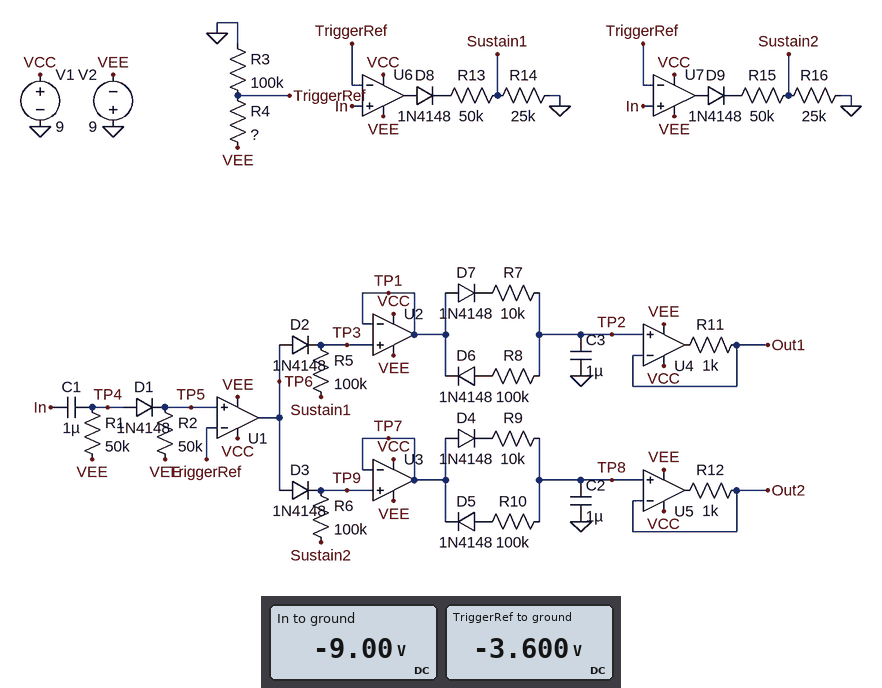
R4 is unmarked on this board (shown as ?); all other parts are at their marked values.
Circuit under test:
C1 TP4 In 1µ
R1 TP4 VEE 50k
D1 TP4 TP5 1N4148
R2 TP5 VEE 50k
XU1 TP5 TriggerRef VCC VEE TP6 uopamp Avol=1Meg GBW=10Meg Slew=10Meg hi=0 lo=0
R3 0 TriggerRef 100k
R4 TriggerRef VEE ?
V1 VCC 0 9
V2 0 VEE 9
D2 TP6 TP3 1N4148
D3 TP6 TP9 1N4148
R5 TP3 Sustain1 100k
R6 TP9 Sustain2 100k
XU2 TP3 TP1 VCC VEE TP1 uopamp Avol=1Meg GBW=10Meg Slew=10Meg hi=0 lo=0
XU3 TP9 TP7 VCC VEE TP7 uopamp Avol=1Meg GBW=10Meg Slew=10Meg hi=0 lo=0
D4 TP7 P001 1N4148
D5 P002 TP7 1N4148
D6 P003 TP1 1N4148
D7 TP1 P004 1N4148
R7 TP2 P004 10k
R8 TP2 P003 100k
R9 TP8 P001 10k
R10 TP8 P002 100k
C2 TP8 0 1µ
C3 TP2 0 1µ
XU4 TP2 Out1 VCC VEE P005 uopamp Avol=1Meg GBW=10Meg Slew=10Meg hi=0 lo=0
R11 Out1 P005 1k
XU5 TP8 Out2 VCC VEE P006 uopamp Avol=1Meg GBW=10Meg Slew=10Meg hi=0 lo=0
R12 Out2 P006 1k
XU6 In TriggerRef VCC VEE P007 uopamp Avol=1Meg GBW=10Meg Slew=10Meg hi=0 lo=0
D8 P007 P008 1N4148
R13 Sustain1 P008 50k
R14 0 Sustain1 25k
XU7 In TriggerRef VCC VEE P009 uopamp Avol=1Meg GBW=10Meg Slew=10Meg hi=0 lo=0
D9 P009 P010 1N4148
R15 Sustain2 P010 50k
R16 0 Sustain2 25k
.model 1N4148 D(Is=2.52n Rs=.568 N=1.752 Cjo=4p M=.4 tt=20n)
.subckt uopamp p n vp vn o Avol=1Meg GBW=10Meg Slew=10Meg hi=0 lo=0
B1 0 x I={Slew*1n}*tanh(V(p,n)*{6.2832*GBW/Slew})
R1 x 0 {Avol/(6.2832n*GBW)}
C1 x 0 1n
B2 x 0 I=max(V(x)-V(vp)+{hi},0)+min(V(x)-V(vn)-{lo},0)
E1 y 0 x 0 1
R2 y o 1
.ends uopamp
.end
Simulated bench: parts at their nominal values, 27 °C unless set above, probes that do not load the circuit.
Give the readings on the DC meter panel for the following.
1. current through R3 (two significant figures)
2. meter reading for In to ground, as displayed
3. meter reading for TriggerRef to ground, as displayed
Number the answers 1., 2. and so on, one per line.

1. 36 µA
2. -9.00 V
3. -3.600 V
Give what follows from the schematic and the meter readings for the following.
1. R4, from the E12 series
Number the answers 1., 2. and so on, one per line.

1. 150 kΩ
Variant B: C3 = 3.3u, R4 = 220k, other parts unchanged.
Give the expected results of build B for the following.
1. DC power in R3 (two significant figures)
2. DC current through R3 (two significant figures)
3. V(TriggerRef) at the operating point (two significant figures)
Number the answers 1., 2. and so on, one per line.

1. 79 µW
2. 28 µA
3. -2.8 V
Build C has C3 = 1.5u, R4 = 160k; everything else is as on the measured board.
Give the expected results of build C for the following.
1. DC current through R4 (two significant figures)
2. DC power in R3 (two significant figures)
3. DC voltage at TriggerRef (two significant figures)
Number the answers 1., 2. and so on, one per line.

1. 35 µA
2. 120 µW
3. -3.5 V
